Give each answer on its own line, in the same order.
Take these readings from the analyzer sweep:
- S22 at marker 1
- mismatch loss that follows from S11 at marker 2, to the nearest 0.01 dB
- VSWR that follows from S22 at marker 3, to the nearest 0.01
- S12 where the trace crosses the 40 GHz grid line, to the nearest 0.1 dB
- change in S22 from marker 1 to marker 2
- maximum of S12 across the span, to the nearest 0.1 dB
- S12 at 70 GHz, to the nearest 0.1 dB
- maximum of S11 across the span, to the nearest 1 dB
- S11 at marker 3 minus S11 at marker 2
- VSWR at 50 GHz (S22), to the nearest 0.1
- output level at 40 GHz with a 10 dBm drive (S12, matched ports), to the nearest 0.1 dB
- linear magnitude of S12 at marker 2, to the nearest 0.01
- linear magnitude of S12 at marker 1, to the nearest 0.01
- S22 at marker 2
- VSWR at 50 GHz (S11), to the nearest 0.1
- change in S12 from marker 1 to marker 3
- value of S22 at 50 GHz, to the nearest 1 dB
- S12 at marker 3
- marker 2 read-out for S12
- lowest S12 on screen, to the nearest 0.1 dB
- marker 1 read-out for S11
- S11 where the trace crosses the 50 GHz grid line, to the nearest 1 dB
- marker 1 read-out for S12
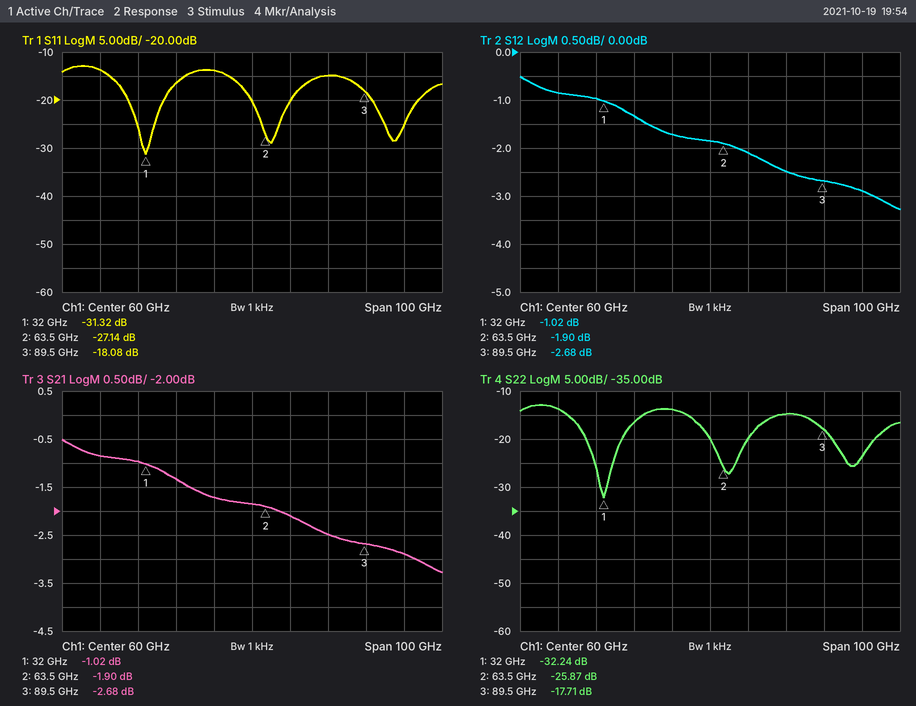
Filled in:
-32.24 dB
0.01 dB
1.30
-1.3 dB
6.37 dB
-0.5 dB
-2.1 dB
-13 dB
9.06 dB
1.5
8.7 dBm
0.80
0.89
-25.87 dB
1.5
-1.66 dB
-14 dB
-2.68 dB
-1.90 dB
-3.3 dB
-31.32 dB
-14 dB
-1.02 dB
